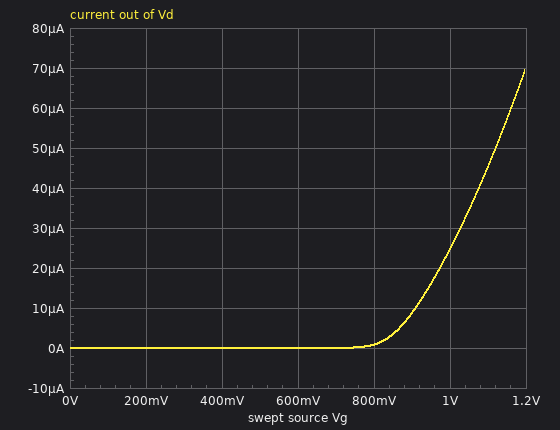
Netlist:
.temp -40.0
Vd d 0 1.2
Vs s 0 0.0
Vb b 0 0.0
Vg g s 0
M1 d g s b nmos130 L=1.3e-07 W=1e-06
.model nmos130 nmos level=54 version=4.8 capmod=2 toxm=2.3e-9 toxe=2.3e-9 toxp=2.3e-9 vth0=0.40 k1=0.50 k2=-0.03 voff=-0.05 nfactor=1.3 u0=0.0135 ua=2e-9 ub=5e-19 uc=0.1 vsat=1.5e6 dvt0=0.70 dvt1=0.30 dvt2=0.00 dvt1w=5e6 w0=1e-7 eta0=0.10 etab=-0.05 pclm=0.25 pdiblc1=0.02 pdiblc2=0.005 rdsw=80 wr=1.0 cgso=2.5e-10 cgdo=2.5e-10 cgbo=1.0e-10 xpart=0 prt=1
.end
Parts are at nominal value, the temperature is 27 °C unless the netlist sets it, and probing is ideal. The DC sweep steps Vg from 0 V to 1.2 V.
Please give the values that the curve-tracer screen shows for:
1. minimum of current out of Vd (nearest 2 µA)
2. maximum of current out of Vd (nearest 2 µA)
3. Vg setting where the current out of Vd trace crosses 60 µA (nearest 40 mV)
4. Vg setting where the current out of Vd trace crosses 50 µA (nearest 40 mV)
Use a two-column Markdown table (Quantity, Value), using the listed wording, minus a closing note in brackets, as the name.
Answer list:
| Quantity | Value |
|---|---|
| minimum of current out of Vd | 0 A |
| maximum of current out of Vd | 70 µA |
| Vg setting where the current out of Vd trace crosses 60 µA | 1.16 V |
| Vg setting where the current out of Vd trace crosses 50 µA | 1.12 V |
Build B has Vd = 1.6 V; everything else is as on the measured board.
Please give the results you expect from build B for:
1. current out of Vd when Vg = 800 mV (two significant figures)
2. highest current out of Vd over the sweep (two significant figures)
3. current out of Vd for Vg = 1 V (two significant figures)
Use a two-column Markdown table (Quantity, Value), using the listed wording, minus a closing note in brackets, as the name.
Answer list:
| Quantity | Value |
|---|---|
| current out of Vd when Vg = 800 mV | 1.0 µA |
| highest current out of Vd over the sweep | 72 µA |
| current out of Vd for Vg = 1 V | 26 µA |
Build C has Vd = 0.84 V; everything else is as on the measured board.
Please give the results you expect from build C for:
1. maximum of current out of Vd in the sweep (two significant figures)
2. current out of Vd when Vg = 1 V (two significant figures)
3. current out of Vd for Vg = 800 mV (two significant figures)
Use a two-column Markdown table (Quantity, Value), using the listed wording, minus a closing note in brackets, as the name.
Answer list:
| Quantity | Value |
|---|---|
| maximum of current out of Vd in the sweep | 68 µA |
| current out of Vd when Vg = 1 V | 24 µA |
| current out of Vd for Vg = 800 mV | 770 nA |
